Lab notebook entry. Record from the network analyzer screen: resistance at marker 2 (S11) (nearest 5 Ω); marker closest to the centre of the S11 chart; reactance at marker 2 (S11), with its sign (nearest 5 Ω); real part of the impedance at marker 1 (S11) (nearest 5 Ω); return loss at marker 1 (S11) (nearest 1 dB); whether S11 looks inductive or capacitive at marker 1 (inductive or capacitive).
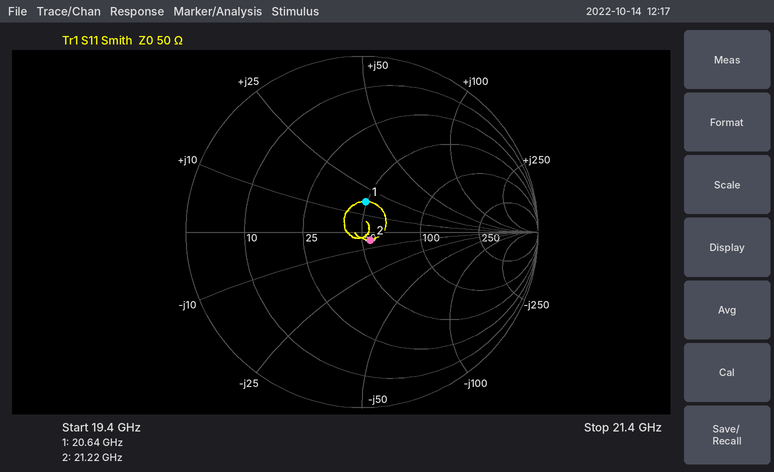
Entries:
55 Ω
marker 2
-5 Ω
50 Ω
15 dB
inductive
